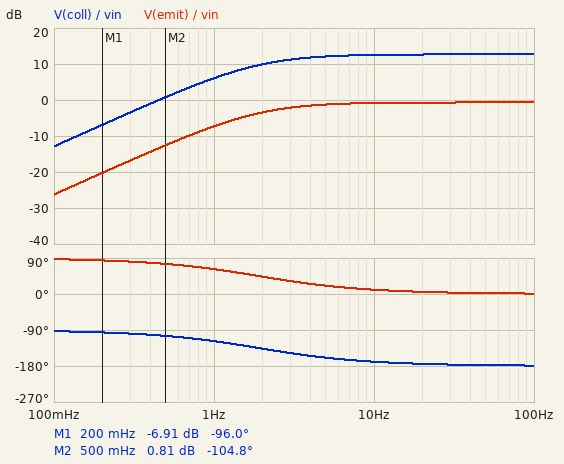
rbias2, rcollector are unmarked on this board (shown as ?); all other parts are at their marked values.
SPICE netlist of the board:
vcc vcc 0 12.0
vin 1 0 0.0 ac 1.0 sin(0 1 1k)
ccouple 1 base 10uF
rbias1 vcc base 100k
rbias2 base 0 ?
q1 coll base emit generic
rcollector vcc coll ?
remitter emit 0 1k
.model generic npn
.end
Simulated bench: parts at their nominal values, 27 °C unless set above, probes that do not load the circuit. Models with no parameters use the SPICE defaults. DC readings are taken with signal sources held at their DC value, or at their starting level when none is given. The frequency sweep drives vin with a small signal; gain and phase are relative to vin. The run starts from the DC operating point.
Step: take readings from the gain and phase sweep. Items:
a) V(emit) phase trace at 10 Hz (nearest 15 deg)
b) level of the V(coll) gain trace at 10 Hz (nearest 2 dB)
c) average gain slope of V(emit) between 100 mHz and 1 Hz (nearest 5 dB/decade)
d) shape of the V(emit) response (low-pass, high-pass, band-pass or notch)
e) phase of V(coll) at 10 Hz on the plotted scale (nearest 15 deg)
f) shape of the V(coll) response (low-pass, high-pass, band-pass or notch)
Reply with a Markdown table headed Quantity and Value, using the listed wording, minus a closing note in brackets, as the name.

| Quantity | Value |
|---|---|
| V(emit) phase trace at 10 Hz | 15 deg |
| level of the V(coll) gain trace at 10 Hz | 12 dB |
| average gain slope of V(emit) between 100 mHz and 1 Hz | 20 dB/decade |
| shape of the V(emit) response | high-pass |
| phase of V(coll) at 10 Hz on the plotted scale | -165 deg |
| shape of the V(coll) response | high-pass |
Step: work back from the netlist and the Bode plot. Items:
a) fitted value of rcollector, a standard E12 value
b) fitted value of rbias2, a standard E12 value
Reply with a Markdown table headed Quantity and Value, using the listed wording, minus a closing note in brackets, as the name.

| Quantity | Value |
|---|---|
| fitted value of rcollector, a standard E12 value | 4.7 kΩ |
| fitted value of rbias2, a standard E12 value | 10 kΩ |
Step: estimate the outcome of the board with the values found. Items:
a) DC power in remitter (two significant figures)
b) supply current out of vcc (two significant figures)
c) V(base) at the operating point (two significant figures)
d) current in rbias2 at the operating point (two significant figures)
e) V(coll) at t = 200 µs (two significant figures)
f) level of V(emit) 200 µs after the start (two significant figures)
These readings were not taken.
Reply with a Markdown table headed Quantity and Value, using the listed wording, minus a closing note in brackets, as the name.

| Quantity | Value |
|---|---|
| DC power in remitter | 100 µW |
| supply current out of vcc | 420 µA |
| V(base) at the operating point | 1.1 V |
| current in rbias2 at the operating point | 110 µA |
| V(coll) at t = 200 µs | 6.3 V |
| level of V(emit) 200 µs after the start | 1.2 V |
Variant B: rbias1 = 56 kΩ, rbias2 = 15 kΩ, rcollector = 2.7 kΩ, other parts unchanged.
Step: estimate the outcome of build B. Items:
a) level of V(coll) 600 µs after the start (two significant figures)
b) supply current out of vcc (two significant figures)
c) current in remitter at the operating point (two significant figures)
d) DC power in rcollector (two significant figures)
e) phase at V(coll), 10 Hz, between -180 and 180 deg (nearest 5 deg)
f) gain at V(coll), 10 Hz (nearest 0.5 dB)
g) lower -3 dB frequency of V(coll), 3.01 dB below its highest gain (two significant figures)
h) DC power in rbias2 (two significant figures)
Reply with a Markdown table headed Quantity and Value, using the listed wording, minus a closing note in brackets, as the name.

| Quantity | Value |
|---|---|
| level of V(coll) 600 µs after the start | 9.4 V |
| supply current out of vcc | 1.7 mA |
| current in remitter at the operating point | 1.6 mA |
| DC power in rcollector | 6.5 mW |
| phase at V(coll), 10 Hz, between -180 and 180 deg | -170 deg |
| gain at V(coll), 10 Hz | 8.5 dB |
| lower -3 dB frequency of V(coll), 3.01 dB below its highest gain | 1.5 Hz |
| DC power in rbias2 | 370 µW |
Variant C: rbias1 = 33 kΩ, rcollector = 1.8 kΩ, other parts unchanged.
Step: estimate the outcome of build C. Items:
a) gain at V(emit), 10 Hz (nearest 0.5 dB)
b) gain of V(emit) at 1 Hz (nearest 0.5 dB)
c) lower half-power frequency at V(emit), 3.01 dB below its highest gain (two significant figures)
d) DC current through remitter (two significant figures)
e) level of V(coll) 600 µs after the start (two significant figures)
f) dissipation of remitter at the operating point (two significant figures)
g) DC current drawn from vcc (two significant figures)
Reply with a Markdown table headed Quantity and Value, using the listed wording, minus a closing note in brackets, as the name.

| Quantity | Value |
|---|---|
| gain at V(emit), 10 Hz | -0.5 dB |
| gain of V(emit) at 1 Hz | -8.0 dB |
| lower half-power frequency at V(emit), 3.01 dB below its highest gain | 2.2 Hz |
| DC current through remitter | 1.9 mA |
| level of V(coll) 600 µs after the start | 9.7 V |
| dissipation of remitter at the operating point | 3.5 mW |
| DC current drawn from vcc | 2.1 mA |
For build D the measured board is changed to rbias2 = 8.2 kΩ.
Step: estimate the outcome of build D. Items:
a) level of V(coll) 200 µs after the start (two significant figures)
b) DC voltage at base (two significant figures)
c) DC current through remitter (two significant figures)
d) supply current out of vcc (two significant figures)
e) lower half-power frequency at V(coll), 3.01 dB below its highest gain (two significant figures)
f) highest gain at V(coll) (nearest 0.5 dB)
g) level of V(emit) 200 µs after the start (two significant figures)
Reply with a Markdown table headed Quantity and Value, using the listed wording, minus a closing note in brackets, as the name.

| Quantity | Value |
|---|---|
| level of V(coll) 200 µs after the start | 7.0 V |
| DC voltage at base | 900 mV |
| DC current through remitter | 170 µA |
| supply current out of vcc | 280 µA |
| lower half-power frequency at V(coll), 3.01 dB below its highest gain | 2.2 Hz |
| highest gain at V(coll) | 12.0 dB |
| level of V(emit) 200 µs after the start | 1.1 V |
